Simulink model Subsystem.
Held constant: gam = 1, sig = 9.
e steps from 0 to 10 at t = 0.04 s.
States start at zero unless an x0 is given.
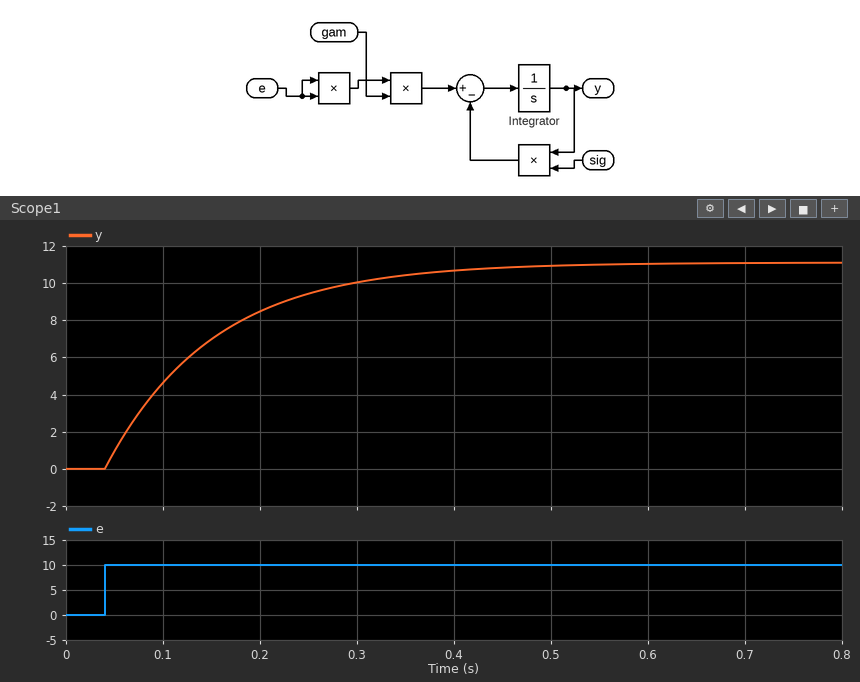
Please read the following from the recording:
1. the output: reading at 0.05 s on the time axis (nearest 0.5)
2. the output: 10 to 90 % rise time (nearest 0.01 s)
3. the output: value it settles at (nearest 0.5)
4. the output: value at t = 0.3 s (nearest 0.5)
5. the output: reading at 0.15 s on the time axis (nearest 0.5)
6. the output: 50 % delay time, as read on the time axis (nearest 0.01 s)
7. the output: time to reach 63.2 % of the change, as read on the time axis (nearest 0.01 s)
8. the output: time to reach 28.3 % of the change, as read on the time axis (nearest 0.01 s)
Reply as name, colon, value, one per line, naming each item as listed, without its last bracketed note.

the output: reading at 0.05 s on the time axis: 1.0
the output: 10 to 90 % rise time: 0.24 s
the output: value it settles at: 11.0
the output: value at t = 0.3 s: 10.0
the output: reading at 0.15 s on the time axis: 7.0
the output: 50 % delay time, as read on the time axis: 0.12 s
the output: time to reach 63.2 % of the change, as read on the time axis: 0.15 s
the output: time to reach 28.3 % of the change, as read on the time axis: 0.08 s
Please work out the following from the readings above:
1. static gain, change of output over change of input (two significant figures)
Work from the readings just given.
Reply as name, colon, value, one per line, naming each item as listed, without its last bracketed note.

static gain, change of output over change of input: 1.1
